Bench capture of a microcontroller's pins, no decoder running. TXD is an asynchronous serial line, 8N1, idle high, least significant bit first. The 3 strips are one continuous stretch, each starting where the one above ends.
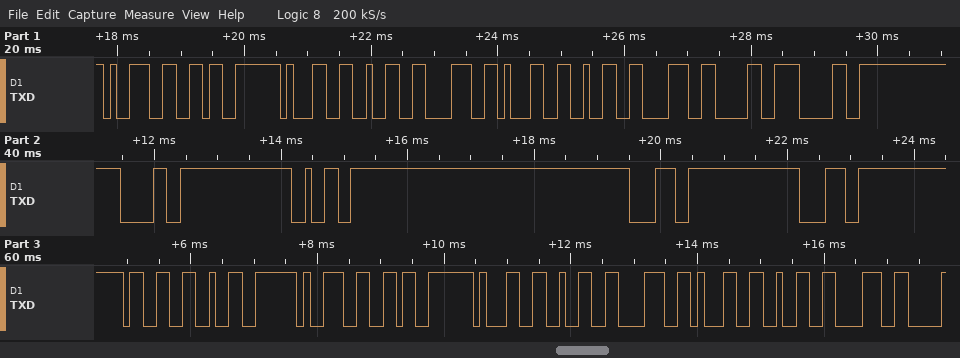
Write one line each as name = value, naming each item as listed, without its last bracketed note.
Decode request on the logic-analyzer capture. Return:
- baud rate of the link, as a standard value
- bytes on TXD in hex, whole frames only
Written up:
baud rate of the link, as a standard value = 9600 baud
bytes on TXD in hex, whole frames only = 39 36 31 32 38 31 32 38 30 30 30 32 38 38 33 32 39 36 31 32 38 31 32 38
